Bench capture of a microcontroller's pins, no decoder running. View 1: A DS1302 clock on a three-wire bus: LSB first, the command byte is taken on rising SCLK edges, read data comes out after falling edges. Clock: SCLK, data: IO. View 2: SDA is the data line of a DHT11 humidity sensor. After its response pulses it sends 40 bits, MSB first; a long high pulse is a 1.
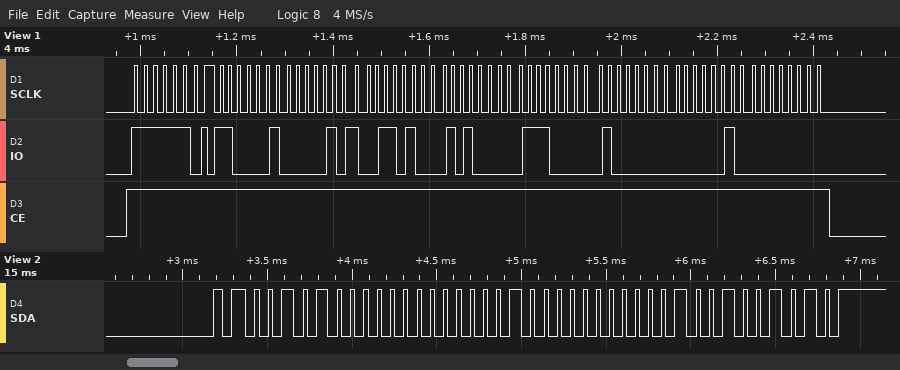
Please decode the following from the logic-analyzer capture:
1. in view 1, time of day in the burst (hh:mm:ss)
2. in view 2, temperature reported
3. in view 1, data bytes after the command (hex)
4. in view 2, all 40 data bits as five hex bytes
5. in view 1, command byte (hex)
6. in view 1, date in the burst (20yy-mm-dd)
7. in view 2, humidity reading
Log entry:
16:50:43
32.2 °C
43 50 16 05 07 01 20 00
28 00 20 02 4A
0xBF
2020-07-05
40 %
